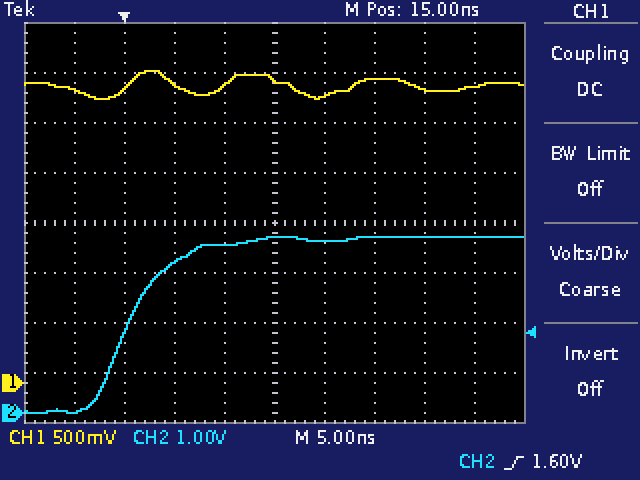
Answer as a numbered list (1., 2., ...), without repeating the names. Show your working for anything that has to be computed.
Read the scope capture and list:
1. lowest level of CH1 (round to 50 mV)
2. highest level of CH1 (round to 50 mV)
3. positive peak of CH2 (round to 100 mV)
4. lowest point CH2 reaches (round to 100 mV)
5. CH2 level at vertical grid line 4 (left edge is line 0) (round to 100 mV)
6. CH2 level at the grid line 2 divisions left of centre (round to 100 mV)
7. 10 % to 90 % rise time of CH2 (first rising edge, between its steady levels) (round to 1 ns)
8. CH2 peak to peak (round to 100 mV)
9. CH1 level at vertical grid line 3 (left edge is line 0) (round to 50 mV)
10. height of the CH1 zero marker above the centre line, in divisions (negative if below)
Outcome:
1. 2.85 V
2. 3.10 V
3. 3.5 V
4. 0.0 V
5. 3.4 V
6. 3.0 V
7. 9 ns
8. 3.5 V − (0.0 V) = 3.5 V
9. 3.00 V
10. -3.2 div
